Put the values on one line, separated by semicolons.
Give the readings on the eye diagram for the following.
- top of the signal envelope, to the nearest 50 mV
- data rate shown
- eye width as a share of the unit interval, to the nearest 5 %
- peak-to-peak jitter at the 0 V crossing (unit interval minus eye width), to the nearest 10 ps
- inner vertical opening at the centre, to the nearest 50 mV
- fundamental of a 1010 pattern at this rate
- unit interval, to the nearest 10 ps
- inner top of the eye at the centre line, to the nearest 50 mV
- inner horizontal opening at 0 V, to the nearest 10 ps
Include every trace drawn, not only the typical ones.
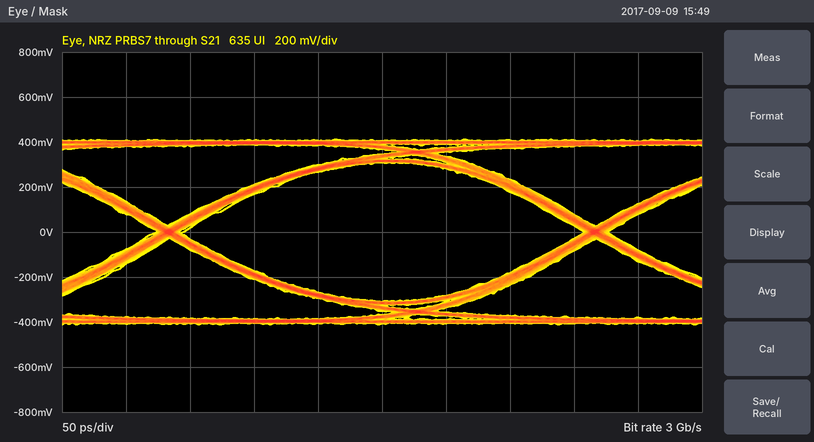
400 mV; 3 Gb/s; 95 %; 20 ps; 600 mV; 1.5 GHz; 330 ps; 300 mV; 310 ps
